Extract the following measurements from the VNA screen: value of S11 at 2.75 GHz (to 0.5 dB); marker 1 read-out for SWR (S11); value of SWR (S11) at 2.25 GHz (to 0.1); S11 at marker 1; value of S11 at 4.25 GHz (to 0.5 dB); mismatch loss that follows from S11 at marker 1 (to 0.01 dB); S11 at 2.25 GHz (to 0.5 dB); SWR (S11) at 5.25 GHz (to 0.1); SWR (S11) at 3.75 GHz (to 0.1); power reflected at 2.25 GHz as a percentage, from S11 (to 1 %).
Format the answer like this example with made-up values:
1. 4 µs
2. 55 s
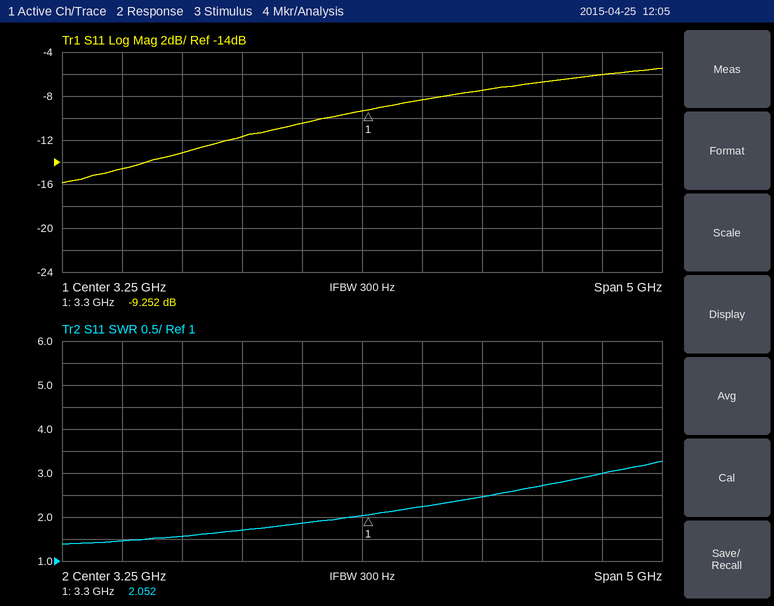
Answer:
1. -10.5 dB
2. 2.052
3. 1.7
4. -9.252 dB
5. -7.5 dB
6. 0.55 dB
7. -11.5 dB
8. 3.0
9. 2.2
10. 7 %
